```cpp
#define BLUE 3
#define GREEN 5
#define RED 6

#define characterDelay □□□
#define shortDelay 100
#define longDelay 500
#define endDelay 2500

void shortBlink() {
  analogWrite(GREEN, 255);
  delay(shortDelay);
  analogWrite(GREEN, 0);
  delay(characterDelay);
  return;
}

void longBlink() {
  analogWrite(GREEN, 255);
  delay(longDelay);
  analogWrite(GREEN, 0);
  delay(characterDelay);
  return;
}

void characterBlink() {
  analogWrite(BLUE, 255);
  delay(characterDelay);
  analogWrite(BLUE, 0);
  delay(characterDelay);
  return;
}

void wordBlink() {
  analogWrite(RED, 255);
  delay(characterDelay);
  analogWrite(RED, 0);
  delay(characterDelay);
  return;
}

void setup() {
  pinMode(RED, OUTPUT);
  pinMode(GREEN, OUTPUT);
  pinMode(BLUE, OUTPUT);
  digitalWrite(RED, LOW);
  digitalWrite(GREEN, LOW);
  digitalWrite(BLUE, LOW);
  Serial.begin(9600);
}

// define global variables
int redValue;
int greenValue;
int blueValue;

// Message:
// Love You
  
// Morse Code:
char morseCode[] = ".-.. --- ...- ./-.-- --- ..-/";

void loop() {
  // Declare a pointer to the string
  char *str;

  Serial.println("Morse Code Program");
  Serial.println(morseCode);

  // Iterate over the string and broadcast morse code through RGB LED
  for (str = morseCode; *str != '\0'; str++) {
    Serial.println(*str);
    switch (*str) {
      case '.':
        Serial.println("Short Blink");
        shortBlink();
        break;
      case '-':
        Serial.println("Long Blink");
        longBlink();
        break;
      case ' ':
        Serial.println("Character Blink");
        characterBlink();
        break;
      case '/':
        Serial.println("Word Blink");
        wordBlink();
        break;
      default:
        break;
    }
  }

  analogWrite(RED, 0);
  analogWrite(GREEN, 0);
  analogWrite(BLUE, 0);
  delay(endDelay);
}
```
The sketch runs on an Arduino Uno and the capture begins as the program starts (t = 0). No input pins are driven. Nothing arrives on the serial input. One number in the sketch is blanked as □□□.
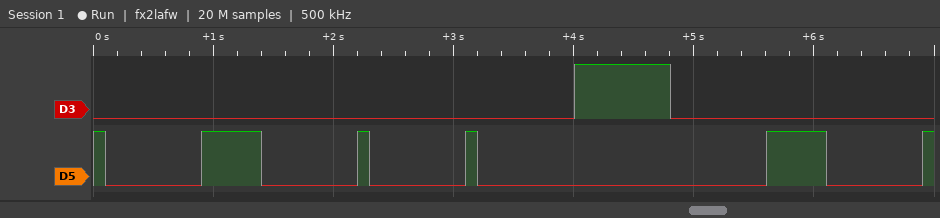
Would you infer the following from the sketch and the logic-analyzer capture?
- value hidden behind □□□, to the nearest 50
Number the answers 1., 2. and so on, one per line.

1. 800
